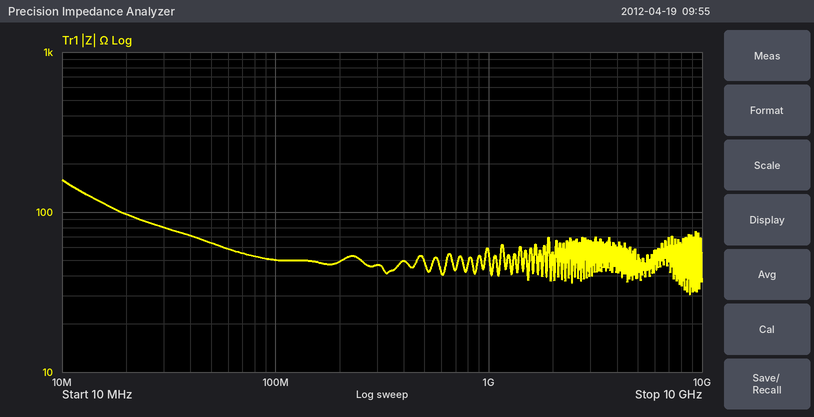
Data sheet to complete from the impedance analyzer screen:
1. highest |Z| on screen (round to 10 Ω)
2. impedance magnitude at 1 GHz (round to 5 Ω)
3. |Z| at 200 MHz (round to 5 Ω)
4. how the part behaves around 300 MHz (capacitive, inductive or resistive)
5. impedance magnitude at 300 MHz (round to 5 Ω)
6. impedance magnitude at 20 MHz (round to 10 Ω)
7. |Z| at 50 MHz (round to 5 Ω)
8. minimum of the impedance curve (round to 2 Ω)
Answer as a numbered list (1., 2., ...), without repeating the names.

1. 160 Ω
2. 55 Ω
3. 50 Ω
4. resistive
5. 45 Ω
6. 100 Ω
7. 65 Ω
8. 30 Ω
